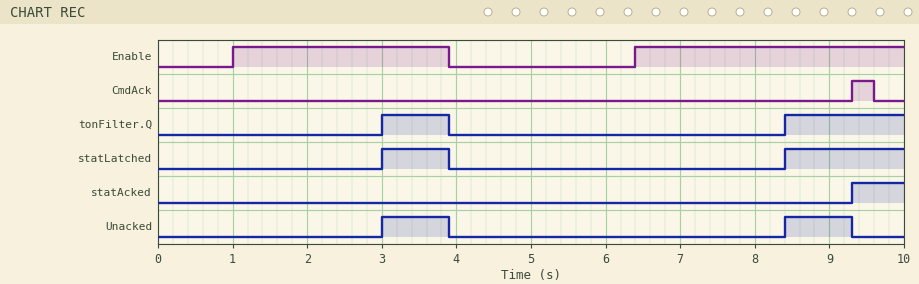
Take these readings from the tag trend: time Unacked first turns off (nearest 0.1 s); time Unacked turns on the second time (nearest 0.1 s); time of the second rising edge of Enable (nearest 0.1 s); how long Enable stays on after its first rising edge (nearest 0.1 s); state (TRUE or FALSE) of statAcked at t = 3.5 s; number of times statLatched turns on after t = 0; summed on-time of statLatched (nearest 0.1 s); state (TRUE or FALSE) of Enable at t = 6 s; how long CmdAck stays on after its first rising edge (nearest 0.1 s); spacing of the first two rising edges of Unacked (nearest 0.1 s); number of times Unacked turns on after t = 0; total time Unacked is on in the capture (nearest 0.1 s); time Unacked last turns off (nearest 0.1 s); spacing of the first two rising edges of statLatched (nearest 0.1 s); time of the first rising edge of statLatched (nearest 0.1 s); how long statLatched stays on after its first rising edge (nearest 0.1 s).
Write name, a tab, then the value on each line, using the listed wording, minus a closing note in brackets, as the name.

time Unacked first turns off	3.9 s
time Unacked turns on the second time	8.4 s
time of the second rising edge of Enable	6.4 s
how long Enable stays on after its first rising edge	2.9 s
state (TRUE or FALSE) of statAcked at t = 3.5 s	FALSE
number of times statLatched turns on after t = 0	2
summed on-time of statLatched	2.5 s
state (TRUE or FALSE) of Enable at t = 6 s	FALSE
how long CmdAck stays on after its first rising edge	0.3 s
spacing of the first two rising edges of Unacked	5.4 s
number of times Unacked turns on after t = 0	2
total time Unacked is on in the capture	1.8 s
time Unacked last turns off	9.3 s
spacing of the first two rising edges of statLatched	5.4 s
time of the first rising edge of statLatched	3.0 s
how long statLatched stays on after its first rising edge	0.9 s
